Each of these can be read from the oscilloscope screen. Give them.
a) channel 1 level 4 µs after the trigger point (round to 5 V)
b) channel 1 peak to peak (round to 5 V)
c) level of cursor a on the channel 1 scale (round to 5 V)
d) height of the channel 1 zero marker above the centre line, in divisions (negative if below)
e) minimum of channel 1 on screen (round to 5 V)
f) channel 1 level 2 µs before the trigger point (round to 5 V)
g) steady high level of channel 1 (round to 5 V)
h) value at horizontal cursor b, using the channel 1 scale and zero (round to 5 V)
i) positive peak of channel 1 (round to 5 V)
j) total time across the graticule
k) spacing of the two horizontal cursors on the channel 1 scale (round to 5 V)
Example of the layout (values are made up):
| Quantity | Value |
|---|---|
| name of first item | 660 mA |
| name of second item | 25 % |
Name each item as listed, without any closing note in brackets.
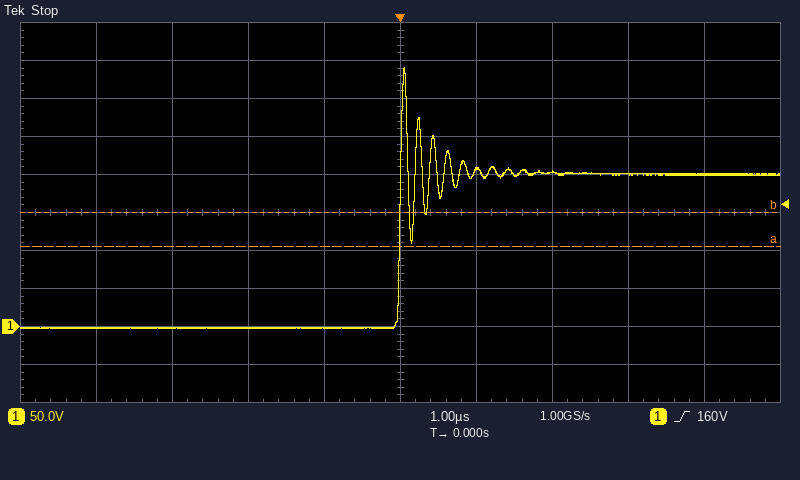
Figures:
| Quantity | Value |
|---|---|
| channel 1 level 4 µs after the trigger point | 200 V |
| channel 1 peak to peak | 345 V |
| level of cursor a on the channel 1 scale | 105 V |
| height of the channel 1 zero marker above the centre line, in divisions | -3.0 div |
| minimum of channel 1 on screen | -5 V |
| channel 1 level 2 µs before the trigger point | 0 V |
| steady high level of channel 1 | 200 V |
| value at horizontal cursor b, using the channel 1 scale and zero | 150 V |
| positive peak of channel 1 | 340 V |
| total time across the graticule | 10 µs |
| spacing of the two horizontal cursors on the channel 1 scale | 45 V |
